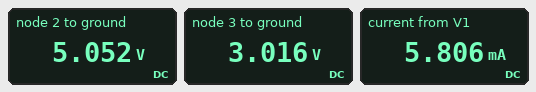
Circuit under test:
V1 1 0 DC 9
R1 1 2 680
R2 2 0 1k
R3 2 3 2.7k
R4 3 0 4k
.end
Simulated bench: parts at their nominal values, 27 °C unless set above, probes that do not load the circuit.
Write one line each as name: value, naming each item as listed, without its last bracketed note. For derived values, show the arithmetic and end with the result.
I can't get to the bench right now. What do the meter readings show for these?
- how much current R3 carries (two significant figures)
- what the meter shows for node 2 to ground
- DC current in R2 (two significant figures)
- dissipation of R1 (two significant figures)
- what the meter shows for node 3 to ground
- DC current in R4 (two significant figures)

how much current R3 carries: (5.052 V - 3.016 V) / 2.7 kΩ = 750 µA
what the meter shows for node 2 to ground: 5.052 V
DC current in R2: (5.052 V) / 1 kΩ = 5.1 mA
dissipation of R1: (9 V - 5.052 V)^2 / 680 Ω = 23 mW
what the meter shows for node 3 to ground: 3.016 V
DC current in R4: (3.016 V) / 4 kΩ = 750 µA
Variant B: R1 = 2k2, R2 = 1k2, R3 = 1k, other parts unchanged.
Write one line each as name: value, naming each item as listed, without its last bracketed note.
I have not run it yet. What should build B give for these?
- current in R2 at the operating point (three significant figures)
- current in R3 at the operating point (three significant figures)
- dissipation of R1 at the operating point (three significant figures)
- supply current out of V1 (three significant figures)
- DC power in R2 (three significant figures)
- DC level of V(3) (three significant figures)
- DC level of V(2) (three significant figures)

current in R2 at the operating point: 2.29 mA
current in R3 at the operating point: 550 µA
dissipation of R1 at the operating point: 17.8 mW
supply current out of V1: 2.84 mA
DC power in R2: 6.30 mW
DC level of V(3): 2.20 V
DC level of V(2): 2.75 V
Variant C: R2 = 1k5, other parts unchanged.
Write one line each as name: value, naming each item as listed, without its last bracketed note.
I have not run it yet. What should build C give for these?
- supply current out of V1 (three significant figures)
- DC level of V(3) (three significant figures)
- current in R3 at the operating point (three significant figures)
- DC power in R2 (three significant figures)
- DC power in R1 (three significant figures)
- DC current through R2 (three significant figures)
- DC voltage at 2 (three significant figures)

supply current out of V1: 4.72 mA
DC level of V(3): 3.46 V
current in R3 at the operating point: 864 µA
DC power in R2: 22.3 mW
DC power in R1: 15.2 mW
DC current through R2: 3.86 mA
DC voltage at 2: 5.79 V
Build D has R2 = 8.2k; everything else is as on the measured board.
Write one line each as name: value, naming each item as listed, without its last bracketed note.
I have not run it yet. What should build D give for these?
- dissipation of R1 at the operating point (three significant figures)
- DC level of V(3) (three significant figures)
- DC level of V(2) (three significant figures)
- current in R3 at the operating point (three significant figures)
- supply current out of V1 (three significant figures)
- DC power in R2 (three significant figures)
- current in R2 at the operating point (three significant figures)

dissipation of R1 at the operating point: 2.89 mW
DC level of V(3): 4.54 V
DC level of V(2): 7.60 V
current in R3 at the operating point: 1.13 mA
supply current out of V1: 2.06 mA
DC power in R2: 7.04 mW
current in R2 at the operating point: 927 µA
